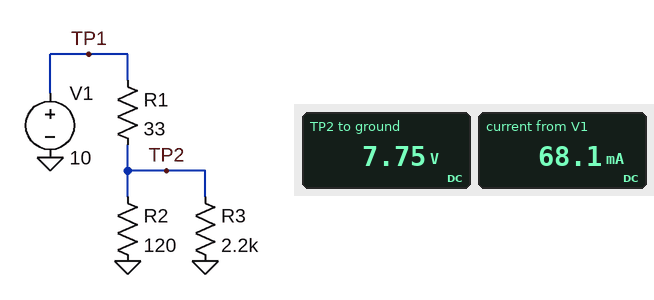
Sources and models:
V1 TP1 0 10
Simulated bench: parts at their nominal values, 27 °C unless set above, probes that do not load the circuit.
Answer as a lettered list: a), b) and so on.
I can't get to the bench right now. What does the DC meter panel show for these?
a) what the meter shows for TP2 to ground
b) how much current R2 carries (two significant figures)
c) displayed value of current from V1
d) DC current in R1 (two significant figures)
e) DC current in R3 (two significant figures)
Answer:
a) 7.75 V
b) 65 mA
c) 68.1 mA
d) 68 mA
e) 3.5 mA
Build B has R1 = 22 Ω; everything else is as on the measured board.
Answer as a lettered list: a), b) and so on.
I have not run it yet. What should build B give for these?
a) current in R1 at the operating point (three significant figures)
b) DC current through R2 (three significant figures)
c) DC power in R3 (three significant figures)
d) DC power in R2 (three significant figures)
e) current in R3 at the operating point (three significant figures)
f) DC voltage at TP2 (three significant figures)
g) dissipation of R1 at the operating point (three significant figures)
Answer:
a) 73.6 mA
b) 69.8 mA
c) 31.9 mW
d) 585 mW
e) 3.81 mA
f) 8.38 V
g) 119 mW
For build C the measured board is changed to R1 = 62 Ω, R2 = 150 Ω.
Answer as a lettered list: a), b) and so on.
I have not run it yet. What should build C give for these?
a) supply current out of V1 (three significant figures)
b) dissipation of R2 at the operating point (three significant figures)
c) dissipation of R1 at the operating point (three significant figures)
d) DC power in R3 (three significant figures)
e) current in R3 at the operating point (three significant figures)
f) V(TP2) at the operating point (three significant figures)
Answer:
a) 49.4 mA
b) 321 mW
c) 151 mW
d) 21.9 mW
e) 3.15 mA
f) 6.94 V
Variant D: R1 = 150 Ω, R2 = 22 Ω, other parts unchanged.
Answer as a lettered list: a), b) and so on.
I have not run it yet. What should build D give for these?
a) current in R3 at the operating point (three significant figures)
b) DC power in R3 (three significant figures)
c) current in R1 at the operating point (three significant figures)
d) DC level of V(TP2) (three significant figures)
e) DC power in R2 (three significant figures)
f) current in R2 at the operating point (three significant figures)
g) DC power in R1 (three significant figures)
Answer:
a) 576 µA
b) 731 µW
c) 58.2 mA
d) 1.27 V
e) 73.1 mW
f) 57.6 mA
g) 508 mW
